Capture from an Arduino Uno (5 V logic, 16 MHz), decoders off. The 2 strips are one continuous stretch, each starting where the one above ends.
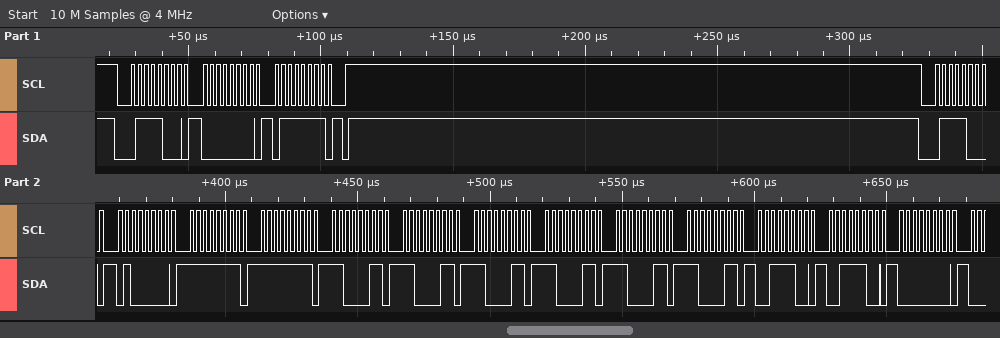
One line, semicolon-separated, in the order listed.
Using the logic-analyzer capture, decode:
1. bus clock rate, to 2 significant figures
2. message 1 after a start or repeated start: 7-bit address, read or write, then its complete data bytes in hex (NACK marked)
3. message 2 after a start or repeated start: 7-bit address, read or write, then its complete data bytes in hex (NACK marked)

400 kHz; 0x3C write: 00 7F; 0x3C write: 40 FF FF C3 C3 C3 C3 C3 C3 3C 3C 00
